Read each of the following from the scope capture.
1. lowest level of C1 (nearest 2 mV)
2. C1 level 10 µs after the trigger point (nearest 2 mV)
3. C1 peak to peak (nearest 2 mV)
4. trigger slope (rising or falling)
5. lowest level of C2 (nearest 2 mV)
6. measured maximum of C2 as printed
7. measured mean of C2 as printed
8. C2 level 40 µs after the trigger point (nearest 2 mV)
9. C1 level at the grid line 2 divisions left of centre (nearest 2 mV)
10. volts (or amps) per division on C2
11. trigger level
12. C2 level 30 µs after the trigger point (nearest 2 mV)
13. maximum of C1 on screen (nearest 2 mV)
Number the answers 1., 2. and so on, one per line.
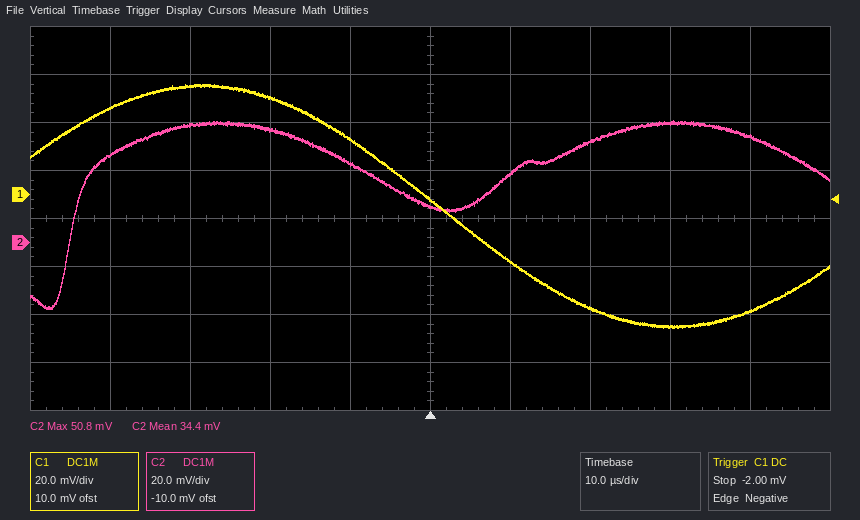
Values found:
1. -56 mV
2. -28 mV
3. 102 mV
4. falling
5. -28 mV
6. 50.8 mV
7. 34.4 mV
8. 44 mV
9. 40 mV
10. 20 mV
11. -2.00 mV
12. 50 mV
13. 46 mV
